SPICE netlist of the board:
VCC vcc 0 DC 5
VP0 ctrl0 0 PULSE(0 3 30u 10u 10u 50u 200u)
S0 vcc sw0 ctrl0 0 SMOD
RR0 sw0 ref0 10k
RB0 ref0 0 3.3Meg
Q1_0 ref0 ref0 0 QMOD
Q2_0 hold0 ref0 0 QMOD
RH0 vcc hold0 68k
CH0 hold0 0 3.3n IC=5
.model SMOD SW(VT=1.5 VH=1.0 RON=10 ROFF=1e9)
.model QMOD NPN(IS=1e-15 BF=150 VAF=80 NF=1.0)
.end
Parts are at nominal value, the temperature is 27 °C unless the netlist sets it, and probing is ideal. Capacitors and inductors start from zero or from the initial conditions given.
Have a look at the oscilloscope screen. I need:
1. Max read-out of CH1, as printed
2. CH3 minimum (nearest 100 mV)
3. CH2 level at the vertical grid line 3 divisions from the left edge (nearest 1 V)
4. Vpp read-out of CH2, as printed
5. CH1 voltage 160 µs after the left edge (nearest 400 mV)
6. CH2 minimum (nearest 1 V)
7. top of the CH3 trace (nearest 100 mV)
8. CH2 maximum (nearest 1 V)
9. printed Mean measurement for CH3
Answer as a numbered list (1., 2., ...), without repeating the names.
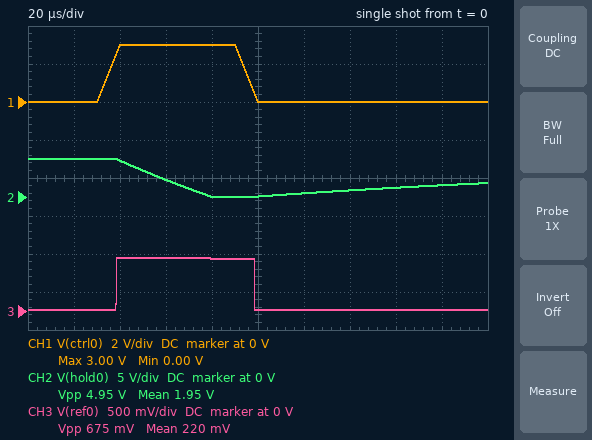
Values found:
1. 3.00 V
2. 0 V
3. 2 V
4. 4.95 V
5. 0 V
6. 0 V
7. 700 mV
8. 5 V
9. 220 mV
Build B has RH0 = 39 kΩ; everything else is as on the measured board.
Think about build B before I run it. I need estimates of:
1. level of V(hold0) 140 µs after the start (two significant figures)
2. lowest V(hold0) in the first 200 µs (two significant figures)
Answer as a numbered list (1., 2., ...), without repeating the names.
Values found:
1. 1.4 V
2. 31 mV
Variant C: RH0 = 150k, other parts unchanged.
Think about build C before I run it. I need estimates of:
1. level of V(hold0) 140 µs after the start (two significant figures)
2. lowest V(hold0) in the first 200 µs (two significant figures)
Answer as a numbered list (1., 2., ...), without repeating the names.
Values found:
1. 420 mV
2. 21 mV
